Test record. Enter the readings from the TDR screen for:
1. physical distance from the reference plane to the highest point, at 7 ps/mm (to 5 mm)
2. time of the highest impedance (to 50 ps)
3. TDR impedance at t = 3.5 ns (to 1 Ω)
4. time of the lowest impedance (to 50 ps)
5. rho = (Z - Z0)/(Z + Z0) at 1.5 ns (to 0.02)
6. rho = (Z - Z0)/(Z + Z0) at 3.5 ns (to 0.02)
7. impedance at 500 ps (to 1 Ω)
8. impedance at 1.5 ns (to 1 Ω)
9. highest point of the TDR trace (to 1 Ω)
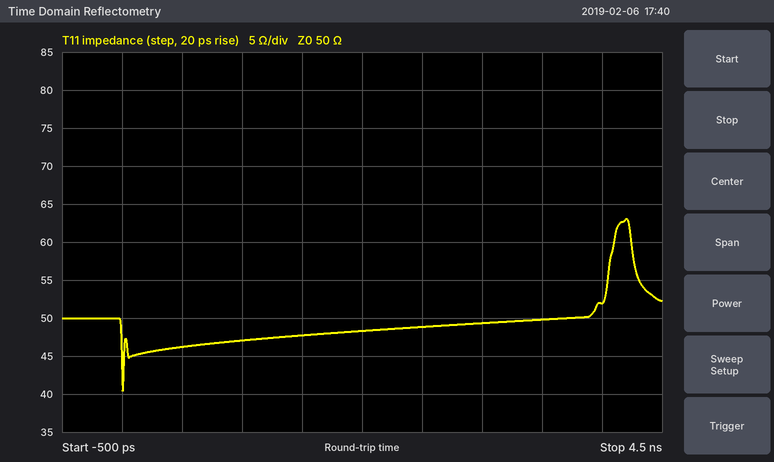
300 mm
4.20 ns
50 Ω
0 ps
-0.02
0.00
46 Ω
48 Ω
63 Ω
